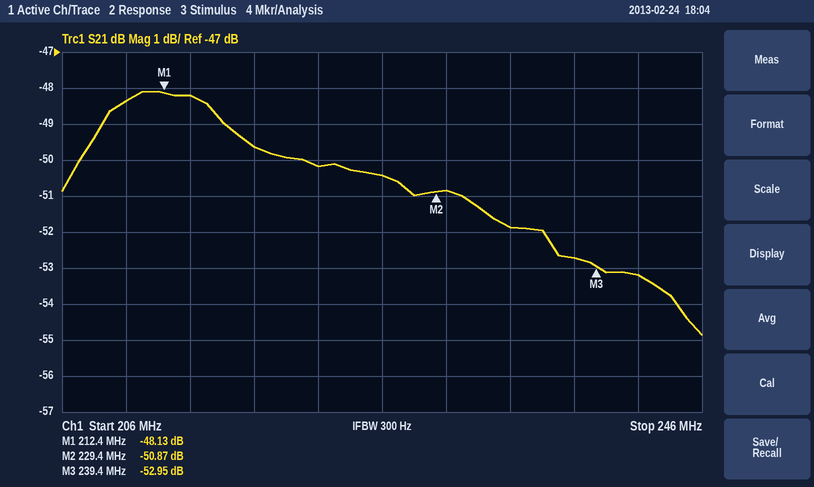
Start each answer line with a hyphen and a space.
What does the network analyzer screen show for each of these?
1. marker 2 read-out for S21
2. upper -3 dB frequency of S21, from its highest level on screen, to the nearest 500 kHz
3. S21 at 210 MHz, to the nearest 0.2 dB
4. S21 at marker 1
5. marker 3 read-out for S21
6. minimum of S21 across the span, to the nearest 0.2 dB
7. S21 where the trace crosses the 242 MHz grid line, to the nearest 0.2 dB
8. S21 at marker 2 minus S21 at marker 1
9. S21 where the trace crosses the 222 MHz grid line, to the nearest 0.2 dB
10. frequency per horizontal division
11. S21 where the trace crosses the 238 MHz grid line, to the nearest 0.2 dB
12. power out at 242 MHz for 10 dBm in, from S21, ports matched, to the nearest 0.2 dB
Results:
- -50.87 dB
- 231.5 MHz
- -48.4 dB
- -48.13 dB
- -52.95 dB
- -54.8 dB
- -53.2 dB
- -2.74 dB
- -50.2 dB
- 4 MHz
- -52.8 dB
- -43.2 dBm
